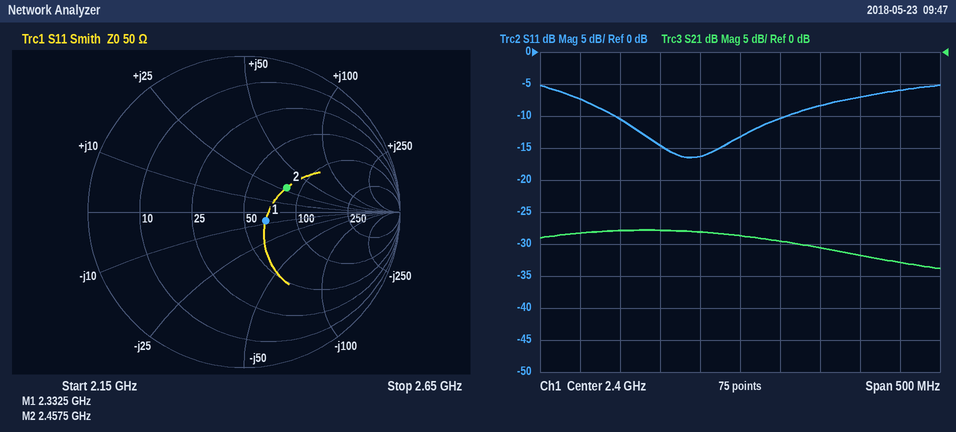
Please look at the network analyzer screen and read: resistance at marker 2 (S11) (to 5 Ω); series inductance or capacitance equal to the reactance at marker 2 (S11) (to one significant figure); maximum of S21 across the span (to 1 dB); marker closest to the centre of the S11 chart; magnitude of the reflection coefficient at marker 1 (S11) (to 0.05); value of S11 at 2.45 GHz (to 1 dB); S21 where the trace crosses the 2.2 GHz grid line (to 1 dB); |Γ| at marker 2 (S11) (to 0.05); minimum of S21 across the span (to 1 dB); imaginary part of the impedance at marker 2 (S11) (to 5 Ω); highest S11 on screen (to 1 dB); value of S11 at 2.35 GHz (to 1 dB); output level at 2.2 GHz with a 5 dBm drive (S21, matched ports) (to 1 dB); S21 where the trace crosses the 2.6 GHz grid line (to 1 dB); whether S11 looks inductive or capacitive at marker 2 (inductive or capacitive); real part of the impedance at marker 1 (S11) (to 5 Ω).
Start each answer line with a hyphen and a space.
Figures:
- 80 Ω
- 2 nH
- -28 dB
- marker 1
- 0.15
- -10 dB
- -28 dB
- 0.30
- -34 dB
- +30 Ω
- -5 dB
- -16 dB
- -23 dBm
- -33 dB
- inductive
- 65 Ω
